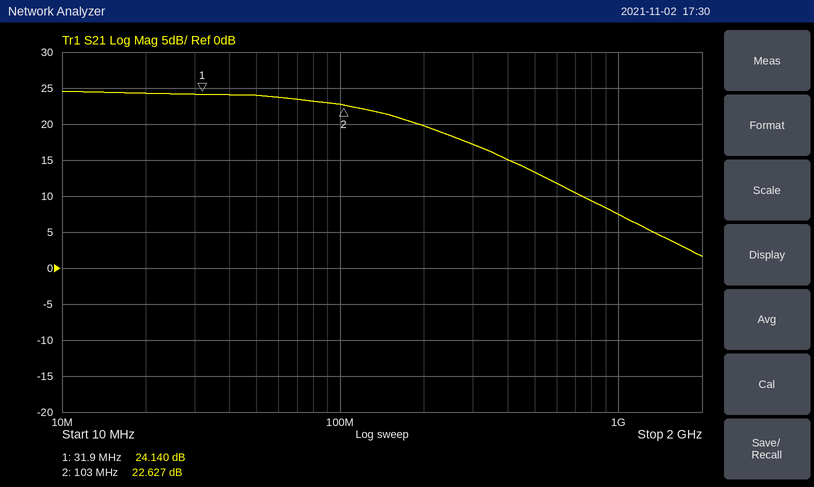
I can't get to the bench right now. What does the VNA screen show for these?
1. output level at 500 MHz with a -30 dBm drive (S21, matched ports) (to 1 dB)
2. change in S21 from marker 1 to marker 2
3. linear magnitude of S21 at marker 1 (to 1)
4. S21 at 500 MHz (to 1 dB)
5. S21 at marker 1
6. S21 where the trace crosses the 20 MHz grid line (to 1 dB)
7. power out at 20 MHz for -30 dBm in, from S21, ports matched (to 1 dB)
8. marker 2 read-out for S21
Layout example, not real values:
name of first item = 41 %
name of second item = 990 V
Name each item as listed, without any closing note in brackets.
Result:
output level at 500 MHz with a -30 dBm drive (S21, matched ports) = -17 dBm
change in S21 from marker 1 to marker 2 = -1.513 dB
linear magnitude of S21 at marker 1 = 16
S21 at 500 MHz = 13 dB
S21 at marker 1 = 24.140 dB
S21 where the trace crosses the 20 MHz grid line = 24 dB
power out at 20 MHz for -30 dBm in, from S21, ports matched = -6 dBm
marker 2 read-out for S21 = 22.627 dB
